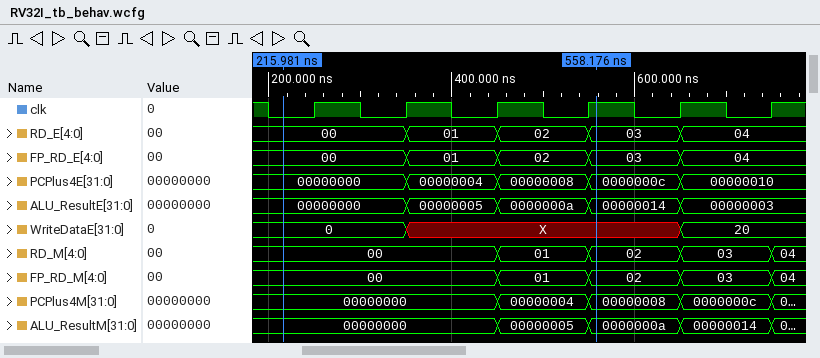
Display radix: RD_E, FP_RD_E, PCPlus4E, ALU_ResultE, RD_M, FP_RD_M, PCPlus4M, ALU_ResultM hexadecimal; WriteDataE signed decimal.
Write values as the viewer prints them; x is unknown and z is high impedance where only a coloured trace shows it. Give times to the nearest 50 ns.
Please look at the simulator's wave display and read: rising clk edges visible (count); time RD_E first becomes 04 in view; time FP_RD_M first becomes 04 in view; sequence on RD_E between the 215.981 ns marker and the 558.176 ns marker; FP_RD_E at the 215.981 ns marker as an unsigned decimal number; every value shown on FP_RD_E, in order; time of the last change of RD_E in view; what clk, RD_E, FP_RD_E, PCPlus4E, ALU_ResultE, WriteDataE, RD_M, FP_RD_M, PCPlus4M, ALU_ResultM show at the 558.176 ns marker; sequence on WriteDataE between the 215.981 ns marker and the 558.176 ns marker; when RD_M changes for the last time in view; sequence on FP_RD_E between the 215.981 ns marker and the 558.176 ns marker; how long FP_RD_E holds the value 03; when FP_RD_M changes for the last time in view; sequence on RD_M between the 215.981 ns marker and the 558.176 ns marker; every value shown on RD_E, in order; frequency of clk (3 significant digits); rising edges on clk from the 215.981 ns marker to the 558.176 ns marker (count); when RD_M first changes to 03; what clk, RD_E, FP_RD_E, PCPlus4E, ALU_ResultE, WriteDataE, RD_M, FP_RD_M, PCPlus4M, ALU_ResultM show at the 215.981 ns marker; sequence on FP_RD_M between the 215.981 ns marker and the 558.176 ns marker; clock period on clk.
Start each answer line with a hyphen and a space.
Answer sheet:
- 6
- 650 ns
- 750 ns
- 00, 01, 02, 03
- 0
- 00, 01, 02, 03, 04
- 650 ns
- clk=1, RD_E=03, FP_RD_E=03, PCPlus4E=0000000c, ALU_ResultE=00000014, WriteDataE=X, RD_M=02, FP_RD_M=02, PCPlus4M=00000008, ALU_ResultM=0000000a
- 0, X
- 750 ns
- 00, 01, 02, 03
- 100 ns
- 750 ns
- 00, 01, 02
- 00, 01, 02, 03, 04
- 10.0 MHz
- 4
- 650 ns
- clk=0, RD_E=00, FP_RD_E=00, PCPlus4E=00000000, ALU_ResultE=00000000, WriteDataE=0, RD_M=00, FP_RD_M=00, PCPlus4M=00000000, ALU_ResultM=00000000
- 00, 01, 02
- 100 ns
